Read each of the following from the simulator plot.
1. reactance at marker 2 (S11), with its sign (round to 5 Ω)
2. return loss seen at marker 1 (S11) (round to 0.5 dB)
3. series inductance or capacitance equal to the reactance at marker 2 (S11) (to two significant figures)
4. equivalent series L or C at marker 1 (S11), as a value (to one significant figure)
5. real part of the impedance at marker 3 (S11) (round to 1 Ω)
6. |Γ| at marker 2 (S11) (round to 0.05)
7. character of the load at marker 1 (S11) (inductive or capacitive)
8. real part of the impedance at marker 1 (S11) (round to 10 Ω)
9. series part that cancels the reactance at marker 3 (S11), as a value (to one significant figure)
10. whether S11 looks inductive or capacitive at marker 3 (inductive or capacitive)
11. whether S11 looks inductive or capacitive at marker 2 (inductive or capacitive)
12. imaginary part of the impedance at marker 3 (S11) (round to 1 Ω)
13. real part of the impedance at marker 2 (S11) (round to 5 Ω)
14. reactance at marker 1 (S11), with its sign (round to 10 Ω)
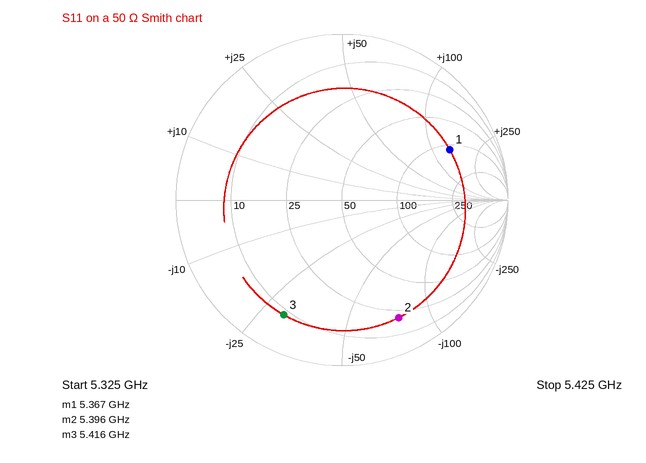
-75 Ω
3.0 dB
390 fF
4 nH
9 Ω
0.80
inductive
110 Ω
900 pH
capacitive
capacitive
-30 Ω
20 Ω
+140 Ω
